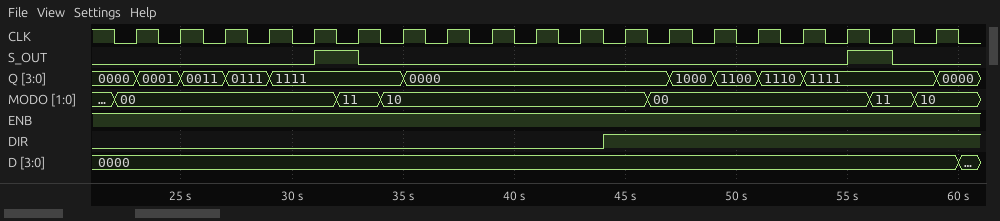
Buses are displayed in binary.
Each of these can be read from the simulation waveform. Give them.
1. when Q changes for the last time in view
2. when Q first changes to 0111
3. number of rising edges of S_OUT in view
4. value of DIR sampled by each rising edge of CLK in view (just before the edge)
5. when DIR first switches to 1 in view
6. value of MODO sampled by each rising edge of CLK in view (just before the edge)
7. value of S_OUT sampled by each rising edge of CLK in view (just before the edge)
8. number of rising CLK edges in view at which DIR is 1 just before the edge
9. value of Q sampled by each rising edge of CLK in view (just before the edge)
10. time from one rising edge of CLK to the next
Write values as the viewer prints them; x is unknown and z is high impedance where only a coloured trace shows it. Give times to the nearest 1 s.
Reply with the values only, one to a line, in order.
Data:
59 s
27 s
2
0 0 0 0 0 0 0 0 0 0 0 1 1 1 1 1 1 1 1
44 s
00, 00, 00, 00, 00, 11, 10, 10, 10, 10, 10, 10, 00, 00, 00, 00, 00, 11, 10
0 0 0 0 0 1 0 0 0 0 0 0 0 0 0 0 0 1 0
8
0000, 0001, 0011, 0111, 1111, 1111, 1111, 0000, 0000, 0000, 0000, 0000, 0000, 1000, 1100, 1110, 1111, 1111, 1111
2 s
